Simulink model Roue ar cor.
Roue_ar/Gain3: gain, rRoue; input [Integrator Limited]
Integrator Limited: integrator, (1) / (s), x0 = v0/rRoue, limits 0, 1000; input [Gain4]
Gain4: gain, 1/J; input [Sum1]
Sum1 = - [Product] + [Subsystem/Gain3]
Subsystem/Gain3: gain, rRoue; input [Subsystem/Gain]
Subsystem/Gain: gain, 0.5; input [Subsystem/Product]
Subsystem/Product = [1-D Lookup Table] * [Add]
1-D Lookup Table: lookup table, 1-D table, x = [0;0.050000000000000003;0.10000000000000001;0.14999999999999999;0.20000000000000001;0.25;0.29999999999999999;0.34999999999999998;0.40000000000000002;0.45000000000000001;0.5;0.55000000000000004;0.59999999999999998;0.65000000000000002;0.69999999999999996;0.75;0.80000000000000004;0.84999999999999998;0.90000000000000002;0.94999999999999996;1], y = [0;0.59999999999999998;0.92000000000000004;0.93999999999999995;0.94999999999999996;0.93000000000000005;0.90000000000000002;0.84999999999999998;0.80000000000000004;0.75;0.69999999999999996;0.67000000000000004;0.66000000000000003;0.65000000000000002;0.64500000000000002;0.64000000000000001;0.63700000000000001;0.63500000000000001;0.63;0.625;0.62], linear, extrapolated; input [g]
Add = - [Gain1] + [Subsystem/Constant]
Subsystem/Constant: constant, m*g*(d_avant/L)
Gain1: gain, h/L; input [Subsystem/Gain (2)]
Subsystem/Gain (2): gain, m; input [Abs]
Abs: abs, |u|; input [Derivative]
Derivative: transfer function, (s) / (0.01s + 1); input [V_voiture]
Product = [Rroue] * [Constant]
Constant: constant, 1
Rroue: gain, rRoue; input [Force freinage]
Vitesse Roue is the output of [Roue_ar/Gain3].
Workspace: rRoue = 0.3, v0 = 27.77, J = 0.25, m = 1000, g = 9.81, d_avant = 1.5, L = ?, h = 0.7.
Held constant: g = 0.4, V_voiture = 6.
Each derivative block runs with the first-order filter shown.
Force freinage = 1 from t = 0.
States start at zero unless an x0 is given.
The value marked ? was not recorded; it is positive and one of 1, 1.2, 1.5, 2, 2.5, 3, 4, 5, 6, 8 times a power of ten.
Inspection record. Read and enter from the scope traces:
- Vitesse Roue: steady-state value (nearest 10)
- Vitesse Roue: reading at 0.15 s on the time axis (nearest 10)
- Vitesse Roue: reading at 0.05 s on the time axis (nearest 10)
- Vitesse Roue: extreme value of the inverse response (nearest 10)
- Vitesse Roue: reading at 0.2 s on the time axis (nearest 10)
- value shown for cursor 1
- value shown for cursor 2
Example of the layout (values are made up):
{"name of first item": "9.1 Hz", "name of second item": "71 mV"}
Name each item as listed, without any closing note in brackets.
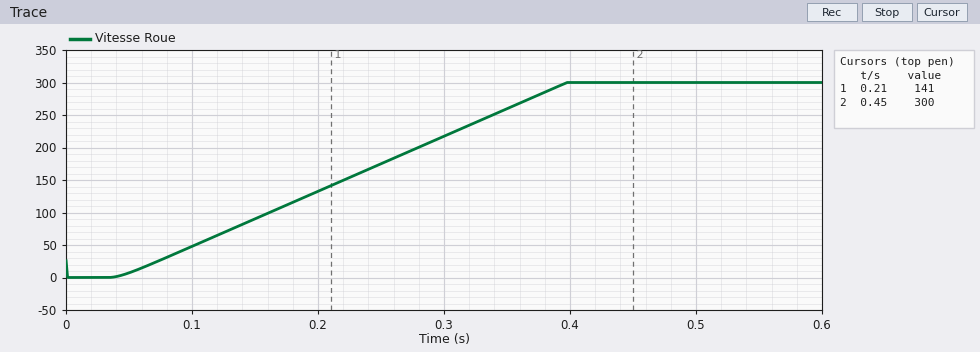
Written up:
{"Vitesse Roue: steady-state value": "300", "Vitesse Roue: reading at 0.15 s on the time axis": "90", "Vitesse Roue: reading at 0.05 s on the time axis": "10", "Vitesse Roue: extreme value of the inverse response": "0", "Vitesse Roue: reading at 0.2 s on the time axis": "130", "value shown for cursor 1": "141", "value shown for cursor 2": "300"}
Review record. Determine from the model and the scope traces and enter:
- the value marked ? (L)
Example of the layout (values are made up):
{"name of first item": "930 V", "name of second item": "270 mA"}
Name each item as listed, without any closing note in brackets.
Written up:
{"the value marked ?": "2.5"}
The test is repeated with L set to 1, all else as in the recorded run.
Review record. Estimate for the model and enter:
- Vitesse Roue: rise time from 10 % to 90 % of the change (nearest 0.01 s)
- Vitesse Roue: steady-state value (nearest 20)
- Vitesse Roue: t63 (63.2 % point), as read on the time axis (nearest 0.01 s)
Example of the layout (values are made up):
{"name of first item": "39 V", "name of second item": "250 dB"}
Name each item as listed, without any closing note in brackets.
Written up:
{"Vitesse Roue: rise time from 10 % to 90 % of the change": "0.10 s", "Vitesse Roue: steady-state value": "300", "Vitesse Roue: t63 (63.2 % point), as read on the time axis": "0.14 s"}
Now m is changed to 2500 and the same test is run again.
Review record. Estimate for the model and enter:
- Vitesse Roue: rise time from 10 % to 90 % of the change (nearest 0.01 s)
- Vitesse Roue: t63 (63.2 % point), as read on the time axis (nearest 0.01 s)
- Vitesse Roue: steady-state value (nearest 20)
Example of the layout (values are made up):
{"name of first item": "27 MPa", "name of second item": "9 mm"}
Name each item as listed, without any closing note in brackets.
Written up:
{"Vitesse Roue: rise time from 10 % to 90 % of the change": "0.10 s", "Vitesse Roue: t63 (63.2 % point), as read on the time axis": "0.14 s", "Vitesse Roue: steady-state value": "300"}
